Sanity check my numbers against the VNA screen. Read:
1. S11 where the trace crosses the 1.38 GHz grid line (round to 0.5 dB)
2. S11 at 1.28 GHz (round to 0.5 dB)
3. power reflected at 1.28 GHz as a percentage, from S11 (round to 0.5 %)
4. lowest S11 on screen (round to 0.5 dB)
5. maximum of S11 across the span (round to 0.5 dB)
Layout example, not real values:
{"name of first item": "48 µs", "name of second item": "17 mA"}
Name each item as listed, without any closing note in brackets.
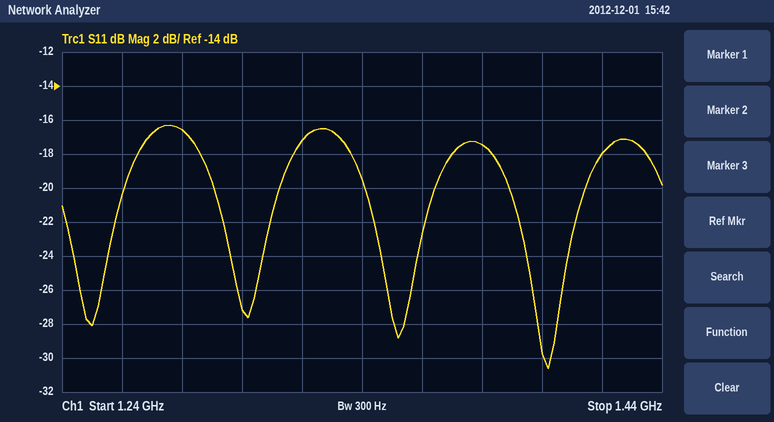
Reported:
{"S11 where the trace crosses the 1.38 GHz grid line": "-17.5 dB", "S11 at 1.28 GHz": "-16.5 dB", "power reflected at 1.28 GHz as a percentage, from S11": "2.0 %", "lowest S11 on screen": "-30.5 dB", "maximum of S11 across the span": "-16.5 dB"}
